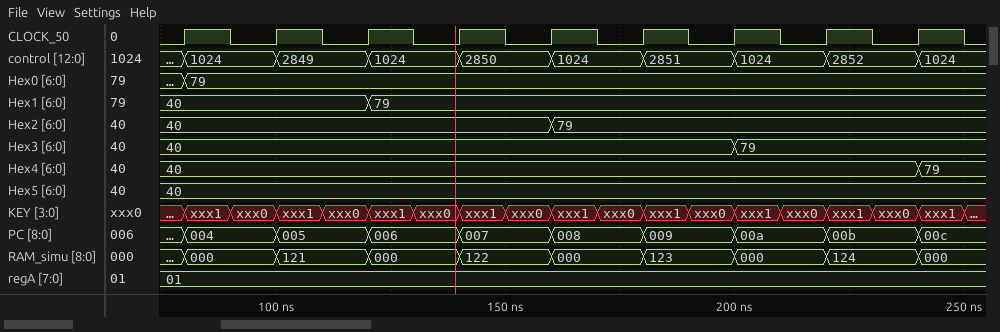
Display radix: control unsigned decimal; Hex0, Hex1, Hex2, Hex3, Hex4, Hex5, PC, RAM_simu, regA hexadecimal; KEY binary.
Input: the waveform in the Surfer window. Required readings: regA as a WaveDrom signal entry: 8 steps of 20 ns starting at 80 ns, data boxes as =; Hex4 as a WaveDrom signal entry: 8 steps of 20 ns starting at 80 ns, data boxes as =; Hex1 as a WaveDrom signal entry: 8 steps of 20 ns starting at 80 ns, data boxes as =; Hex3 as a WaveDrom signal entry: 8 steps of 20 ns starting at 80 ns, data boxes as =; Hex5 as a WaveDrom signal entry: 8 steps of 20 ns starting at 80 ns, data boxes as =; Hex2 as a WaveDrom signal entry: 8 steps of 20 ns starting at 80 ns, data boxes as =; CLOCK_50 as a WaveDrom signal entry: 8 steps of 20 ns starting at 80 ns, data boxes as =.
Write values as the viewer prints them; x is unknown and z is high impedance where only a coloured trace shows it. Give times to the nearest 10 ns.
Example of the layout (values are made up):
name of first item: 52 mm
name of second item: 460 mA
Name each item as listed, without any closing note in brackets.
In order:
regA as a WaveDrom signal entry: 8 steps of 20 ns starting at 80 ns, data boxes as =: {name: 'regA', wave: '=.......', data: '01'}
Hex4 as a WaveDrom signal entry: 8 steps of 20 ns starting at 80 ns, data boxes as =: {name: 'Hex4', wave: '=.......', data: '40'}
Hex1 as a WaveDrom signal entry: 8 steps of 20 ns starting at 80 ns, data boxes as =: {name: 'Hex1', wave: '=.=.....', data: '40 79'}
Hex3 as a WaveDrom signal entry: 8 steps of 20 ns starting at 80 ns, data boxes as =: {name: 'Hex3', wave: '=.....=.', data: '40 79'}
Hex5 as a WaveDrom signal entry: 8 steps of 20 ns starting at 80 ns, data boxes as =: {name: 'Hex5', wave: '=.......', data: '40'}
Hex2 as a WaveDrom signal entry: 8 steps of 20 ns starting at 80 ns, data boxes as =: {name: 'Hex2', wave: '=...=...', data: '40 79'}
CLOCK_50 as a WaveDrom signal entry: 8 steps of 20 ns starting at 80 ns, data boxes as =: {name: 'CLOCK_50', wave: 'p.......'}
